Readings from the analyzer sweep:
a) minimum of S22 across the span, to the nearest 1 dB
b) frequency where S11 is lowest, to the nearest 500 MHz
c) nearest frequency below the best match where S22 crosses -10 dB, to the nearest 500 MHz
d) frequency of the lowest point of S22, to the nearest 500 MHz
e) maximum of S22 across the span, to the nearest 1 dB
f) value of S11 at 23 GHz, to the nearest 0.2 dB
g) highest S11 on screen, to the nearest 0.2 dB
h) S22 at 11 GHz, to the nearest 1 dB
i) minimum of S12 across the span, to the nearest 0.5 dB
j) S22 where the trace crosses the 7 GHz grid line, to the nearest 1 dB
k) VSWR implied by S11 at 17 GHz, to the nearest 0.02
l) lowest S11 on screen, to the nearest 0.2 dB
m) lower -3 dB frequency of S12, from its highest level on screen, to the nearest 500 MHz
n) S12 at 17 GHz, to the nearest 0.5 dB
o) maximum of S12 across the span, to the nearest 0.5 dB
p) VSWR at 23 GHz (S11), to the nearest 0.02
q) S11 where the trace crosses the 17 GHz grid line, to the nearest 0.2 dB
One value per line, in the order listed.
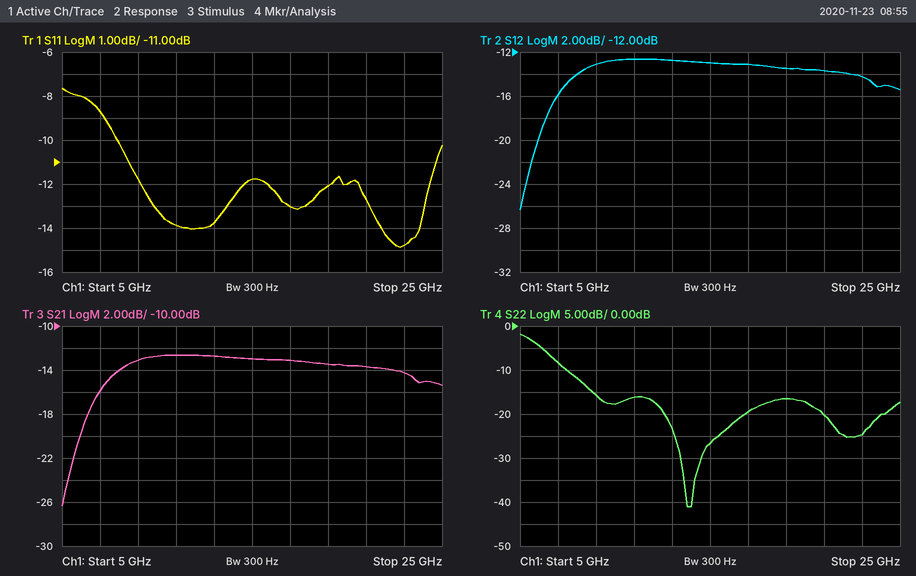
-41 dB
23.0 GHz
7.5 GHz
14.0 GHz
-2 dB
-14.8 dB
-7.6 dB
-16 dB
-26.5 dB
-8 dB
1.58
-14.8 dB
7.0 GHz
-13.0 dB
-12.5 dB
1.44
-13.0 dB
